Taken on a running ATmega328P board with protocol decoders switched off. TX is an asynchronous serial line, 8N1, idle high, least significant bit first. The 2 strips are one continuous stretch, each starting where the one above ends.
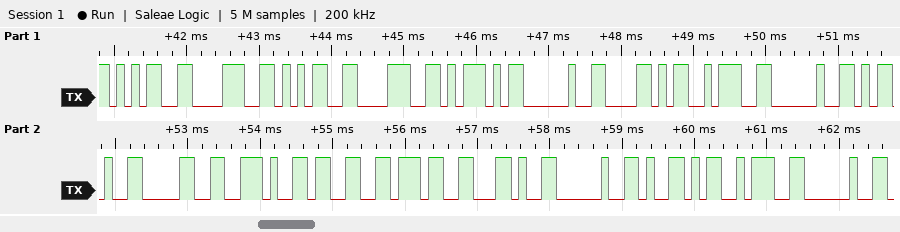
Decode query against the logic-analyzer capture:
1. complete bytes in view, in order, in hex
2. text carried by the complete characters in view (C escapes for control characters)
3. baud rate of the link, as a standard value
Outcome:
35 38 35 38 5D 20 58 3A 20 2D 30 2E 33 37 2C 20 59 3A 20
"5858] X: -0.37, Y: "
9600 baud
